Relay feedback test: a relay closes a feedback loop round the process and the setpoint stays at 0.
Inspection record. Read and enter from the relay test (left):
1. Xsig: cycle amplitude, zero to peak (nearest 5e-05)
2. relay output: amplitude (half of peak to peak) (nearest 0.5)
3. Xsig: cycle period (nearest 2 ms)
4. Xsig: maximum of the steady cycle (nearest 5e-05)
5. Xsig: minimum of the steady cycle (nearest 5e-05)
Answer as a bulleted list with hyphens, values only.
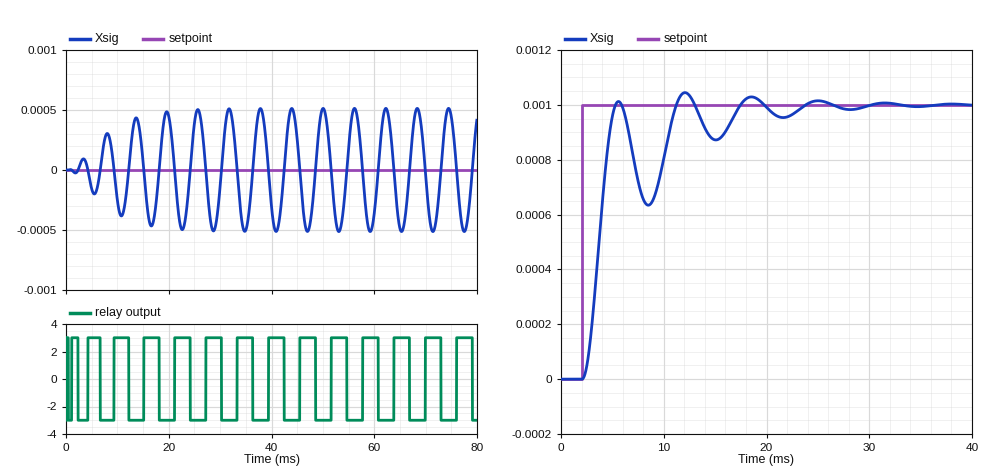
- 0.00050
- 3.0
- 6 ms
- 0.00050
- -0.00050
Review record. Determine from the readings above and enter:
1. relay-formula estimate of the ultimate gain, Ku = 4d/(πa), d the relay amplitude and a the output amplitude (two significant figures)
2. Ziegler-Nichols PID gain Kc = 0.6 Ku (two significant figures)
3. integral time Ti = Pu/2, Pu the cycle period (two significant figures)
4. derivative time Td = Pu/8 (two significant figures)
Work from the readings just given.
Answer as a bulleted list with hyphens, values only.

- 7600
- 4600
- 3.0 ms
- 0.75 ms
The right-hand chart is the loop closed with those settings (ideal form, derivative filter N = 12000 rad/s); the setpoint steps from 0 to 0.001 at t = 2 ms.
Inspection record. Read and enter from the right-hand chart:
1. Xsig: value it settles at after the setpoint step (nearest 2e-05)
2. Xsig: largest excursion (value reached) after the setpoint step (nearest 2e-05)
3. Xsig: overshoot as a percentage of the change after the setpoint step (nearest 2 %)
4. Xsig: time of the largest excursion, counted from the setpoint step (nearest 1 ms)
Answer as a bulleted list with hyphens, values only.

- 0.00100
- 0.00104
- 4 %
- 10 ms
